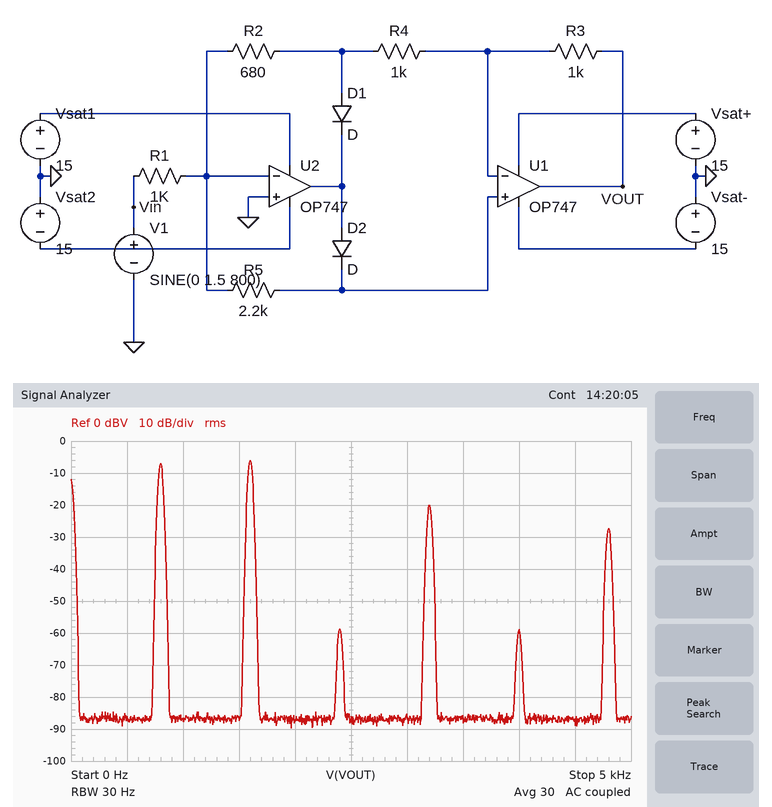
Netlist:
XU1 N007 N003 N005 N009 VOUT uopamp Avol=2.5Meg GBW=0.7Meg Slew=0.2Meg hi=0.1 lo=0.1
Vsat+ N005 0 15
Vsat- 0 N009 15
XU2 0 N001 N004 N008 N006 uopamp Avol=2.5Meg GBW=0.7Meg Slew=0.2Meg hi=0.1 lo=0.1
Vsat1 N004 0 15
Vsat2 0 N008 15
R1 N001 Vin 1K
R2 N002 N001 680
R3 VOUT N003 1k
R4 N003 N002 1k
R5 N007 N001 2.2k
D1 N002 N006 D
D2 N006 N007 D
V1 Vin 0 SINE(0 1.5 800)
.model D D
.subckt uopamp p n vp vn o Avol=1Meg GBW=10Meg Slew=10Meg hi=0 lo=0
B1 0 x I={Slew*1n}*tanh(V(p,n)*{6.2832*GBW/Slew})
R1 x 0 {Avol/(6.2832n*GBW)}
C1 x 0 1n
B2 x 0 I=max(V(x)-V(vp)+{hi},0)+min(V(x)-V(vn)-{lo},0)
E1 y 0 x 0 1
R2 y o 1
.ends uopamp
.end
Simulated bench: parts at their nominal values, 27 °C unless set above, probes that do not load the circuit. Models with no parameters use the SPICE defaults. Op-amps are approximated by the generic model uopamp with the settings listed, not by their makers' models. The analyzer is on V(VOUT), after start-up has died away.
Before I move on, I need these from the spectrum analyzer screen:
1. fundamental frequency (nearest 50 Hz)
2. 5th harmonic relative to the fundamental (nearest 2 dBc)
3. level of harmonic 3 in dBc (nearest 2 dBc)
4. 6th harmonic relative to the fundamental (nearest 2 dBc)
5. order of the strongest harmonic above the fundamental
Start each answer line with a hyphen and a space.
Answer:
- 800 Hz
- -52 dBc
- -52 dBc
- -20 dBc
- 2
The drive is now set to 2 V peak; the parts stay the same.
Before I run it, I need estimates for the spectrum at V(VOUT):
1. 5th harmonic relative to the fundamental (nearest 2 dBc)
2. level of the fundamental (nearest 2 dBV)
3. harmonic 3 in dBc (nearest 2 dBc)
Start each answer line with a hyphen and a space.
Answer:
- -54 dBc
- -4 dBV
- -54 dBc
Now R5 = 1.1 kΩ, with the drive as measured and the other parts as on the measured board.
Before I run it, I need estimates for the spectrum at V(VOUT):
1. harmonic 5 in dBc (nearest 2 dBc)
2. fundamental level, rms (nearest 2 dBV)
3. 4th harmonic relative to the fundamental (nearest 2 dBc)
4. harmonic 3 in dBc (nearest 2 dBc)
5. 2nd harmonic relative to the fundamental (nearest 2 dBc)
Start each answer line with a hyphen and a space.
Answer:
- -46 dBc
- -14 dBV
- -8 dBc
- -46 dBc
- 6 dBc
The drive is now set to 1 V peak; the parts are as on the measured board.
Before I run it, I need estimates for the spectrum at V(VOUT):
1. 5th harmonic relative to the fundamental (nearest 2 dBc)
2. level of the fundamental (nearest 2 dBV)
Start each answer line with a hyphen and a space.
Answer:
- -50 dBc
- -10 dBV
